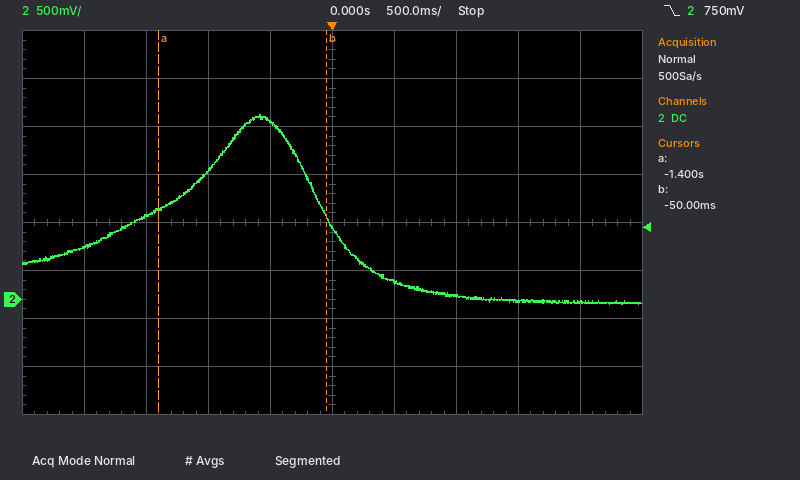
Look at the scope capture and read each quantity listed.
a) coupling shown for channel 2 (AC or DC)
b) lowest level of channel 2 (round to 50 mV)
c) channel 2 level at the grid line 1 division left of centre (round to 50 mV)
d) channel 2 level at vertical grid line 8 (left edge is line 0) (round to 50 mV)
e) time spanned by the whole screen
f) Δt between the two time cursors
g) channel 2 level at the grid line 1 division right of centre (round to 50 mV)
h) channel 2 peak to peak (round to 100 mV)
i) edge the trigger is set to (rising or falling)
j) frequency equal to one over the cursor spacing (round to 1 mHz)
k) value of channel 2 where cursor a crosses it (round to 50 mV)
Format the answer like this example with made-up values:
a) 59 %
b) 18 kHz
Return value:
a) DC
b) -50 mV
c) 1.85 V
d) 0 mV
e) 5 s
f) 1.35 s
g) 200 mV
h) 2.00 V
i) falling
j) 741 mHz
k) 950 mV
